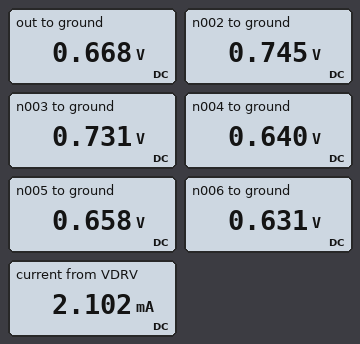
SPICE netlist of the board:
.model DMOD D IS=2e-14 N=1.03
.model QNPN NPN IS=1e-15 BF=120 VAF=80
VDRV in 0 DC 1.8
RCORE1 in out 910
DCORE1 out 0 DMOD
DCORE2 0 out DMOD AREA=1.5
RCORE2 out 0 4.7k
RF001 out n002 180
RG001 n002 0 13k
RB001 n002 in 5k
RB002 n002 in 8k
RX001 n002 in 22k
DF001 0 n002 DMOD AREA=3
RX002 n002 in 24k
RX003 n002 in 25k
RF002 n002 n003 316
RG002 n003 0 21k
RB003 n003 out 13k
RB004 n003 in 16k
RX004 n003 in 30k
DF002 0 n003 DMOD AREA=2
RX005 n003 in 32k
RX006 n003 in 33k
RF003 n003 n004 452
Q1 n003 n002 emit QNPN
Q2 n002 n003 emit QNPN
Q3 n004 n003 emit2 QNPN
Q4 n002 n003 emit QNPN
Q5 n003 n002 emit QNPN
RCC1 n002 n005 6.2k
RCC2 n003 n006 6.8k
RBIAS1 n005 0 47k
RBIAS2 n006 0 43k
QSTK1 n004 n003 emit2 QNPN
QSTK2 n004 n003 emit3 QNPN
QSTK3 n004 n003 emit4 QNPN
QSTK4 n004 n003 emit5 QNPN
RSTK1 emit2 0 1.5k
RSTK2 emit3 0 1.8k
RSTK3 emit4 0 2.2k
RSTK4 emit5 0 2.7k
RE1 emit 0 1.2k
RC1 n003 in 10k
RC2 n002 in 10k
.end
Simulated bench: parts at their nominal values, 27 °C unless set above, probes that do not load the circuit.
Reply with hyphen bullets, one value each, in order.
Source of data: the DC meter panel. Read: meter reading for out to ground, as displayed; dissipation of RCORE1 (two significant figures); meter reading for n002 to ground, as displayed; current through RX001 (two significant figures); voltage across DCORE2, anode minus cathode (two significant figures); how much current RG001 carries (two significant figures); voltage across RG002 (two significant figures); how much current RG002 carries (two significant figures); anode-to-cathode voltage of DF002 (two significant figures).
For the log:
- 0.668 V
- 1.4 mW
- 0.745 V
- 48 µA
- -670 mV
- 57 µA
- 730 mV
- 35 µA
- -730 mV
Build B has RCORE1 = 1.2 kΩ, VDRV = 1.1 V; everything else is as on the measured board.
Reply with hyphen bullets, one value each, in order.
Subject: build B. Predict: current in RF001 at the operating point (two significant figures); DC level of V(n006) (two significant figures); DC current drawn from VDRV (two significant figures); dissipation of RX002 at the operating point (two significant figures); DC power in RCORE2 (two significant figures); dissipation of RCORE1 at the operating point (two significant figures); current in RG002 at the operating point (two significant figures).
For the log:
- 130 µA
- 560 mV
- 750 µA
- 8.2 µW
- 85 µW
- 180 µW
- 31 µA
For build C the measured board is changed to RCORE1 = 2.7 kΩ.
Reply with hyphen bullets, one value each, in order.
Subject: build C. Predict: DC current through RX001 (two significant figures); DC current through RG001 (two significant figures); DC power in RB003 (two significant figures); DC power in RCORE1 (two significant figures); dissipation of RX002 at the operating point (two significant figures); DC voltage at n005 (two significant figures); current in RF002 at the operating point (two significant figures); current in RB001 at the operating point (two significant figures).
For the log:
- 49 µA
- 56 µA
- 440 nW
- 490 µW
- 48 µW
- 650 mV
- 22 µA
- 210 µA
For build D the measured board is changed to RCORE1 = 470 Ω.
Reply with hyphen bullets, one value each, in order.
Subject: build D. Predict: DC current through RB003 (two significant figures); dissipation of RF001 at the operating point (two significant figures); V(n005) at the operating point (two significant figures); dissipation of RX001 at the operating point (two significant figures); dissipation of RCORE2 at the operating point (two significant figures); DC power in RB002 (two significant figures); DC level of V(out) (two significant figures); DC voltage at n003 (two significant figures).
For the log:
- 4.1 µA
- 30 µW
- 670 mV
- 50 µW
- 99 µW
- 140 µW
- 680 mV
- 740 mV
